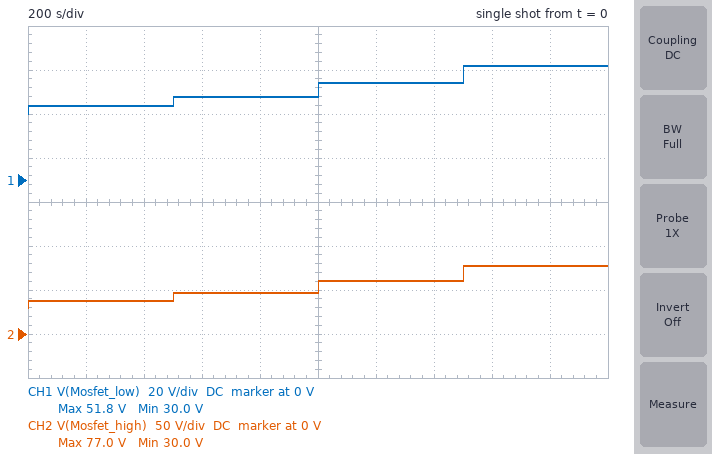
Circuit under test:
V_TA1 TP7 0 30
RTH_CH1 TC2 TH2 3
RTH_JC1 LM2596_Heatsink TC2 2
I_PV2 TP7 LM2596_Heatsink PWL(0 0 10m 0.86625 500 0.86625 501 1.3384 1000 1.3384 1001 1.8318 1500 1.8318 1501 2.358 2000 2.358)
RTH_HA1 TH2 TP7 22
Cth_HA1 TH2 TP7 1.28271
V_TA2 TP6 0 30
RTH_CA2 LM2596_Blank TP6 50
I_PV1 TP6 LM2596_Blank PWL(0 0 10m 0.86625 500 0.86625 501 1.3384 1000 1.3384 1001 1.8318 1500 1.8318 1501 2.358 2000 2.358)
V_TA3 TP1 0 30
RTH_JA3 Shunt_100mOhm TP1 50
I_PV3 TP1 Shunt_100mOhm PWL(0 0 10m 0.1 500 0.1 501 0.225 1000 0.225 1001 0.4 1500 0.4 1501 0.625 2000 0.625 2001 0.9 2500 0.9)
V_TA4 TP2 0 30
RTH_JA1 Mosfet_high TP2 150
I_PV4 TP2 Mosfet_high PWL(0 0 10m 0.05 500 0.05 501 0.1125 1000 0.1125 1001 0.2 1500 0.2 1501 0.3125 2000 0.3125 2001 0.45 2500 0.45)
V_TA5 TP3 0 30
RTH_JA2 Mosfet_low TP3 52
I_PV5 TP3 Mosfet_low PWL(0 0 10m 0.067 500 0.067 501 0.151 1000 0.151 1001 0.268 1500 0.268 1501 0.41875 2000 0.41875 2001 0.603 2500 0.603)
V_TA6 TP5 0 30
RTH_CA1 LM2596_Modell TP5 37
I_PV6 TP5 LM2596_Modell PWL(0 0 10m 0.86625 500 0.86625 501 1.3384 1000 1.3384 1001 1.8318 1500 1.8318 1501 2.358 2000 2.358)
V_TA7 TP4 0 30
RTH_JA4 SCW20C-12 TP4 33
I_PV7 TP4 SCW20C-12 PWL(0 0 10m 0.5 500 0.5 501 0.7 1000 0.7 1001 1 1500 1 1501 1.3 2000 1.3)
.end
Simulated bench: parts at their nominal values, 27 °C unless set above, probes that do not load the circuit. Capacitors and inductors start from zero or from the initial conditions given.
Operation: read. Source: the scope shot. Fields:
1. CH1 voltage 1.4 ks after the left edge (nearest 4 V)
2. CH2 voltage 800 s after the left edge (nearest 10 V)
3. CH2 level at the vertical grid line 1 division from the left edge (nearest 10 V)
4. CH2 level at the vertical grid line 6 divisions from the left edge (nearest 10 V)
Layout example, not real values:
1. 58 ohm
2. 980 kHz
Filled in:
1. 44 V
2. 50 V
3. 40 V
4. 60 V
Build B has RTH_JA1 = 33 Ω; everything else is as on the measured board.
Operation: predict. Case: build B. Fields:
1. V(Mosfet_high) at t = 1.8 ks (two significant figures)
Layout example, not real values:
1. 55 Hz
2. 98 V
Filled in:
1. 40 V
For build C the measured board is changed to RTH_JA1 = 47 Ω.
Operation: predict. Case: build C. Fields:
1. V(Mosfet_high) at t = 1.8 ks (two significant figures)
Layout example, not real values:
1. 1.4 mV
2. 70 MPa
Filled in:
1. 45 V
